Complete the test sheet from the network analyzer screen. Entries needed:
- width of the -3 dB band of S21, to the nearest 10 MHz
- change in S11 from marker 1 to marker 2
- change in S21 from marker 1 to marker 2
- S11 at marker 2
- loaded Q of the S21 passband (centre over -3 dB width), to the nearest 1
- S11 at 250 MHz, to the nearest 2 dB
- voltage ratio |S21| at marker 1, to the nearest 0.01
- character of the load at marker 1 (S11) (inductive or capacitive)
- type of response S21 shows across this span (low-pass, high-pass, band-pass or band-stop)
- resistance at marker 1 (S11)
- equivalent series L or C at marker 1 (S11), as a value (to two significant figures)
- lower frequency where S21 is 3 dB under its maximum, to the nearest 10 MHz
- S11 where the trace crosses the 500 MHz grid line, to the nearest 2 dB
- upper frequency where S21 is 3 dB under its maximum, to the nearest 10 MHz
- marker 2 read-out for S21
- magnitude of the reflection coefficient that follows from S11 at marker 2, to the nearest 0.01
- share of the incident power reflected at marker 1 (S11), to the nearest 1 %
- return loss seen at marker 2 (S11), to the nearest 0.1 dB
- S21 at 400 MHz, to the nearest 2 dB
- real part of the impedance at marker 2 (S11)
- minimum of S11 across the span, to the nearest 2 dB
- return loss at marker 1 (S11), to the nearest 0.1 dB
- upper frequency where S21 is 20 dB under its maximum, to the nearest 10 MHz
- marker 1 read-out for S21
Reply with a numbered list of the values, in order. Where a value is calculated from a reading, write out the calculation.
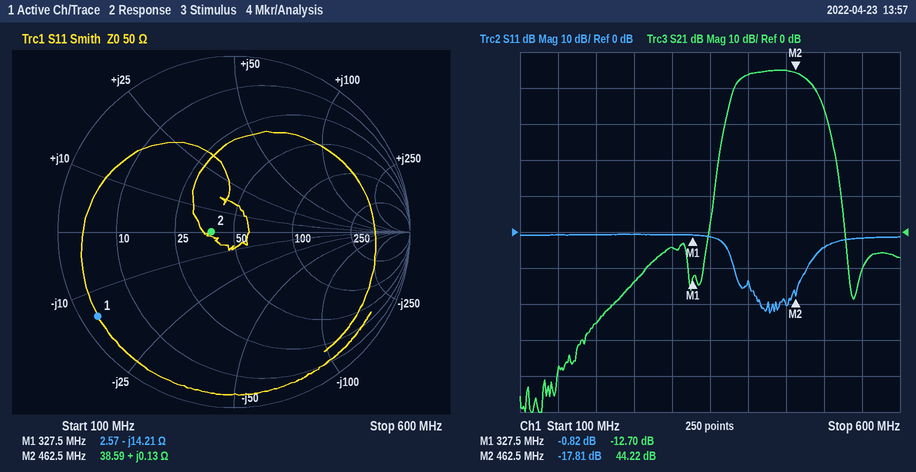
1. 480 MHz − 390 MHz = 90 MHz
2. -17.81 − (-0.82) = -16.99 dB
3. 44.22 − (-12.7) = 56.92 dB
4. -17.81 dB
5. 435 MHz / 90 MHz ≈ 5
6. 0 dB
7. 10^(-12.7/20) ≈ 0.23
8. capacitive
9. band-pass
10. 2.57 Ω
11. C = 1/(2π × 327.5 MHz × 14.21 Ω) ≈ 34 pF
12. 390 MHz
13. -4 dB
14. 480 MHz
15. 44.22 dB
16. 10^(-17.81/20) ≈ 0.13
17. 10^(-0.82/10) ≈ 83 %
18. 17.8 dB
19. 44 dB
20. 38.59 Ω
21. -22 dB
22. 0.8 dB
23. 510 MHz
24. -12.70 dB
